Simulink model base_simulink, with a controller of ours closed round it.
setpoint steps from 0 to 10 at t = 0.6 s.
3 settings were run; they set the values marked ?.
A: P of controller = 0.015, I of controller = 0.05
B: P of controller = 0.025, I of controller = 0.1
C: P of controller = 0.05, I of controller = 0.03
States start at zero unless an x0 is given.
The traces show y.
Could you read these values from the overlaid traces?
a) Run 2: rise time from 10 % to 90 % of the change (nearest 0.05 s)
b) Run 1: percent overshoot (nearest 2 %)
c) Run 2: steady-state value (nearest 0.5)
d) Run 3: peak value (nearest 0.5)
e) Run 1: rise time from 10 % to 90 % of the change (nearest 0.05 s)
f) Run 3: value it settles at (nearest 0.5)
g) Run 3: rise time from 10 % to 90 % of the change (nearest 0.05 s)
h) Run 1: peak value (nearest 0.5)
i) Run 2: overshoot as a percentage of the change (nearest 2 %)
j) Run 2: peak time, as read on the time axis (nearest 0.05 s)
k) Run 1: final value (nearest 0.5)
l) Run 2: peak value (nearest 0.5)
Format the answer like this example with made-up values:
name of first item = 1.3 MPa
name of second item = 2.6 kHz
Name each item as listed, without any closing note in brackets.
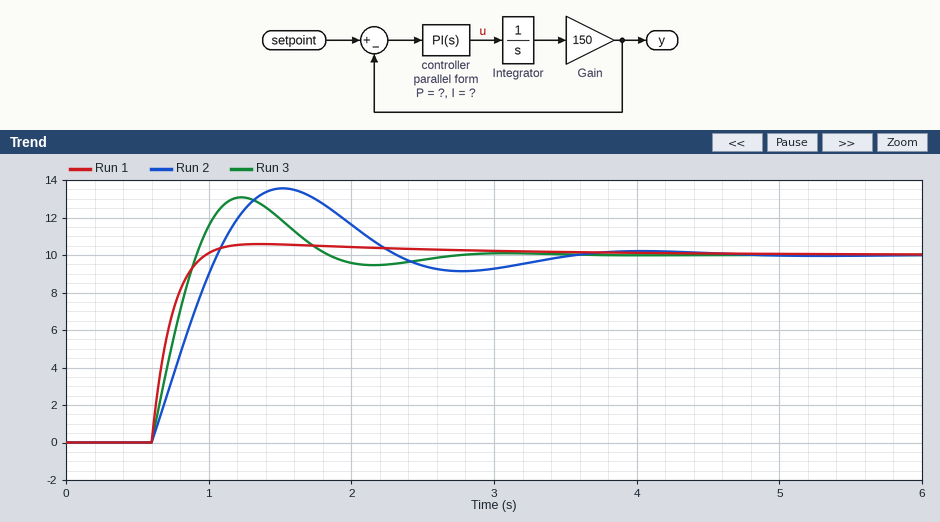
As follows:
Run 2: rise time from 10 % to 90 % of the change = 0.35 s
Run 1: percent overshoot = 6 %
Run 2: steady-state value = 10.0
Run 3: peak value = 13.0
Run 1: rise time from 10 % to 90 % of the change = 0.25 s
Run 3: value it settles at = 10.0
Run 3: rise time from 10 % to 90 % of the change = 0.25 s
Run 1: peak value = 10.5
Run 2: overshoot as a percentage of the change = 36 %
Run 2: peak time, as read on the time axis = 1.50 s
Run 1: final value = 10.0
Run 2: peak value = 13.5
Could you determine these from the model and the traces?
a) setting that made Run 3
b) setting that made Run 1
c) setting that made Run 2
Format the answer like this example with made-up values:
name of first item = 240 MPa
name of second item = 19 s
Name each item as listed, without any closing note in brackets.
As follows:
setting that made Run 3 = B
setting that made Run 1 = C
setting that made Run 2 = A
